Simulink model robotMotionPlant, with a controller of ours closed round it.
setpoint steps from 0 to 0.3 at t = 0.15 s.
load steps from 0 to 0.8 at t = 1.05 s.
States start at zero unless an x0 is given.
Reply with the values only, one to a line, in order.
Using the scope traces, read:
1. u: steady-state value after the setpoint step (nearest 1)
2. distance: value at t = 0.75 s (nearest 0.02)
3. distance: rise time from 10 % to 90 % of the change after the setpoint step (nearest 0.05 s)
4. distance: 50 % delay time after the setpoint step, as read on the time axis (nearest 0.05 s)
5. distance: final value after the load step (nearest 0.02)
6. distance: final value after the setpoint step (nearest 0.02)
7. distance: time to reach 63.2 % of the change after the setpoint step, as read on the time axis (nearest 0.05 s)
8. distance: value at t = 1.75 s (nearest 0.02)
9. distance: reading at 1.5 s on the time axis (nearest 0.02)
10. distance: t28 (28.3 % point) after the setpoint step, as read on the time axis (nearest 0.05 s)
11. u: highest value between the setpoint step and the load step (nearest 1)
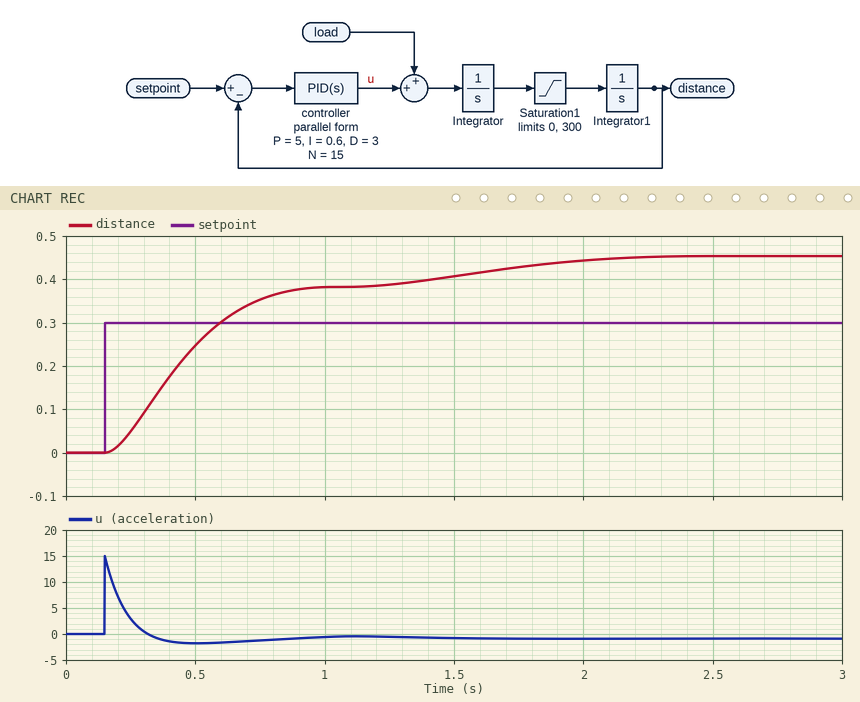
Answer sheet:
-1
0.36
0.50 s
0.40 s
0.46
0.38
0.50 s
0.42
0.40
0.30 s
15
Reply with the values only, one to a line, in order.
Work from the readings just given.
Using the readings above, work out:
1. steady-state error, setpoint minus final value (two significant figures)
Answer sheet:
-0.080
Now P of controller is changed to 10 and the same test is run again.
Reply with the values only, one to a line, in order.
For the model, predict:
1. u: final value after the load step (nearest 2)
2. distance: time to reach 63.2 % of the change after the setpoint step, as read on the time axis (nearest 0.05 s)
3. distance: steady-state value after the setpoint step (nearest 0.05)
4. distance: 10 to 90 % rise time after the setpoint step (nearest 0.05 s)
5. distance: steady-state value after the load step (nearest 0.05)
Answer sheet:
-2
0.45 s
0.40
0.40 s
0.40
